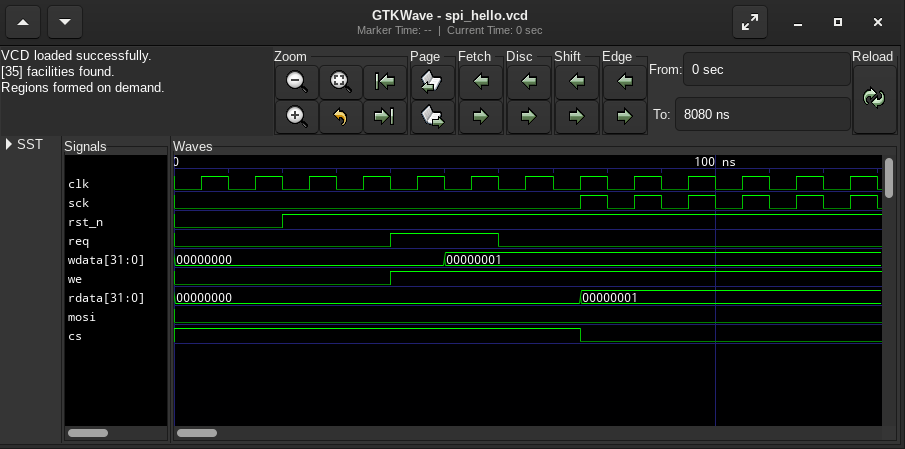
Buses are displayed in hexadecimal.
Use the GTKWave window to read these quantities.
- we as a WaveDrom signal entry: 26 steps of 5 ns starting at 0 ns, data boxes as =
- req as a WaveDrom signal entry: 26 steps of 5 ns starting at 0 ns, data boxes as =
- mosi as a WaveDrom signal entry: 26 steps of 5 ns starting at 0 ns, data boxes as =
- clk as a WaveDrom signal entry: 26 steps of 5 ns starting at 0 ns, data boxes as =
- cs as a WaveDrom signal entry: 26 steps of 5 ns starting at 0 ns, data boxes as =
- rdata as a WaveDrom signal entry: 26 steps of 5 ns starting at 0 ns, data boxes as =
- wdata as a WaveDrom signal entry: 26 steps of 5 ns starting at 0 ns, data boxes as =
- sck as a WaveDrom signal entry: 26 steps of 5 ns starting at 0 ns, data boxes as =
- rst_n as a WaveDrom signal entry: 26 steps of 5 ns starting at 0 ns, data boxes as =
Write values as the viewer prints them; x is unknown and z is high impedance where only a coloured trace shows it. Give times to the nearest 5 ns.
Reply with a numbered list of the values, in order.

1. {name: 'we', wave: '0.......1.................'}
2. {name: 'req', wave: '0.......1...0.............'}
3. {name: 'mosi', wave: '0.........................'}
4. {name: 'clk', wave: '01010101010101010101010101'}
5. {name: 'cs', wave: '1..............0..........'}
6. {name: 'rdata', wave: '=..............=..........', data: '00000000 00000001'}
7. {name: 'wdata', wave: '=.........=...............', data: '00000000 00000001'}
8. {name: 'sck', wave: '0..............10101010101'}
9. {name: 'rst_n', wave: '0...1.....................'}
